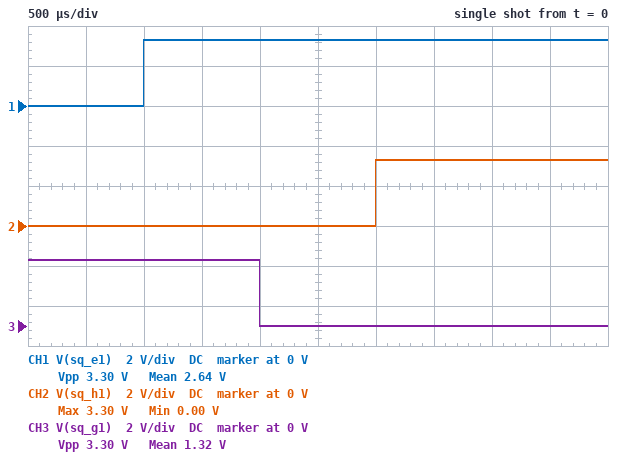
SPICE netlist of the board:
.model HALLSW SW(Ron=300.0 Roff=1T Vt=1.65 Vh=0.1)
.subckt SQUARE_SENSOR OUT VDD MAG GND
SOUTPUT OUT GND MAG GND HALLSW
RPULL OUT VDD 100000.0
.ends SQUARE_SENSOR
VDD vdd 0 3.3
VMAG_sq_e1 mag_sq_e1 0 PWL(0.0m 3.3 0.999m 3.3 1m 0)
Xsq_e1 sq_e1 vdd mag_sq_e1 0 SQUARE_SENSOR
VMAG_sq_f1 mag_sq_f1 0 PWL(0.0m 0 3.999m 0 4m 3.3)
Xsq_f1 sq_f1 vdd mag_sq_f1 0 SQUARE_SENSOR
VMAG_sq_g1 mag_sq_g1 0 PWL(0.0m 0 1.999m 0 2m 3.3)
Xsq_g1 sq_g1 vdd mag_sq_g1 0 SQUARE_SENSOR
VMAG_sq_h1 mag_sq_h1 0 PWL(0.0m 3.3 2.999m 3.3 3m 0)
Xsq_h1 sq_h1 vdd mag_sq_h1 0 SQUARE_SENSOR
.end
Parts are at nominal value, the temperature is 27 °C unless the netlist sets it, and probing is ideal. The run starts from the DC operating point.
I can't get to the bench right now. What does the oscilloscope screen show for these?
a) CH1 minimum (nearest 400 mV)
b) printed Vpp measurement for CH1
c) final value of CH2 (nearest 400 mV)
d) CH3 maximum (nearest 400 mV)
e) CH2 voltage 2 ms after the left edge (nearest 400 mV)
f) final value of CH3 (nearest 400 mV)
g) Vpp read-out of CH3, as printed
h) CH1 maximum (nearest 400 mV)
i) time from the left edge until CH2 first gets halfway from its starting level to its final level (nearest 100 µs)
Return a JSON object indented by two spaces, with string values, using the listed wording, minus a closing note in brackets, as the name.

{
  "CH1 minimum": "0 V",
  "printed Vpp measurement for CH1": "3.30 V",
  "final value of CH2": "3.2 V",
  "CH3 maximum": "3.2 V",
  "CH2 voltage 2 ms after the left edge": "0 V",
  "final value of CH3": "0 V",
  "Vpp read-out of CH3, as printed": "3.30 V",
  "CH1 maximum": "3.2 V",
  "time from the left edge until CH2 first gets halfway from its starting level to its final level": "3.0 ms"
}
